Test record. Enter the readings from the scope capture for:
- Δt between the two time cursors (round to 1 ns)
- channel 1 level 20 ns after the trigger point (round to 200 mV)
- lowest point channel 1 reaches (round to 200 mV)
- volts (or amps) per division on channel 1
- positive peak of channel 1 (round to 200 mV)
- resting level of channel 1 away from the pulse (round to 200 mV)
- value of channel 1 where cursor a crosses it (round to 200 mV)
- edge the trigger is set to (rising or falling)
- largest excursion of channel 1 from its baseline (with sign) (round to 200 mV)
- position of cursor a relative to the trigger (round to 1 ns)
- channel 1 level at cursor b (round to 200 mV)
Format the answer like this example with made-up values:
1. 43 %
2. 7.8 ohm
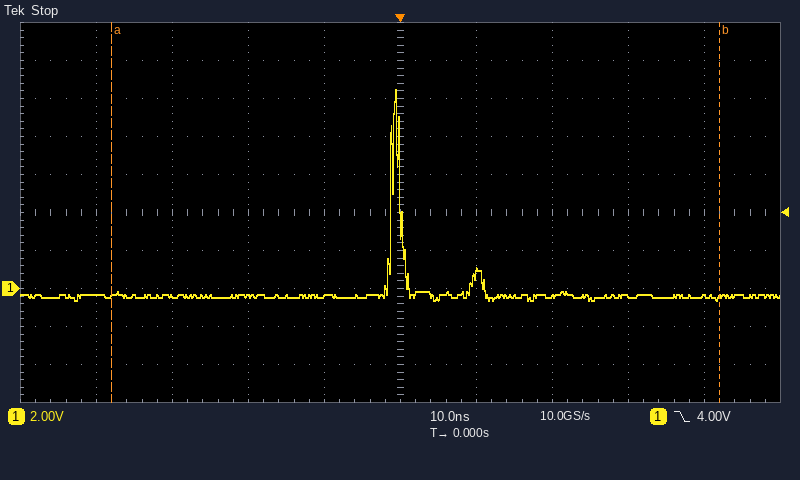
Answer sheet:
1. 80 ns
2. -400 mV
3. -600 mV
4. 2 V
5. 10.4 V
6. -400 mV
7. -400 mV
8. falling
9. +10.8 V
10. -38 ns
11. -400 mV
